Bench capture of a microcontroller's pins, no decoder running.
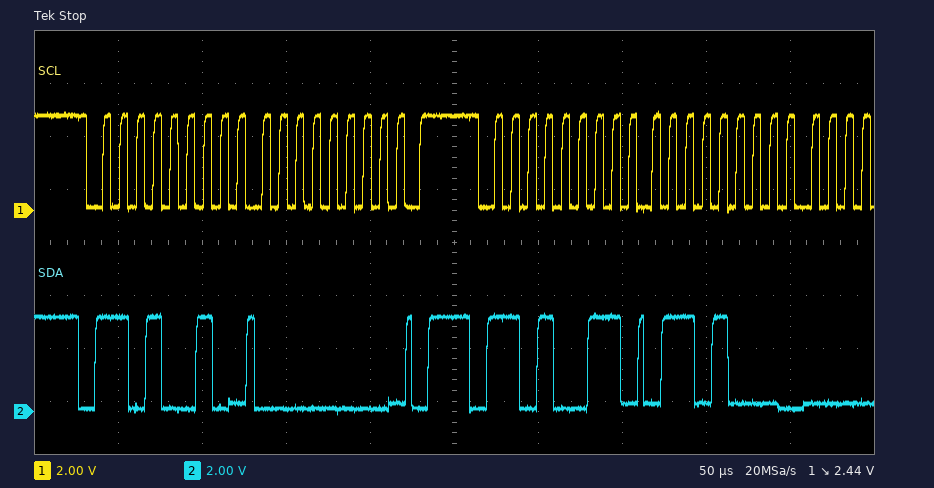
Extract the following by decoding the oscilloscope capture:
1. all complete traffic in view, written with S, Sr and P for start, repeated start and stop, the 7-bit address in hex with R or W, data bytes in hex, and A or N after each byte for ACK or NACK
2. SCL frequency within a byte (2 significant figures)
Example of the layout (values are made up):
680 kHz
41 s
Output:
S 69W A 00 A P S 69R A 68 A
100 kHz
